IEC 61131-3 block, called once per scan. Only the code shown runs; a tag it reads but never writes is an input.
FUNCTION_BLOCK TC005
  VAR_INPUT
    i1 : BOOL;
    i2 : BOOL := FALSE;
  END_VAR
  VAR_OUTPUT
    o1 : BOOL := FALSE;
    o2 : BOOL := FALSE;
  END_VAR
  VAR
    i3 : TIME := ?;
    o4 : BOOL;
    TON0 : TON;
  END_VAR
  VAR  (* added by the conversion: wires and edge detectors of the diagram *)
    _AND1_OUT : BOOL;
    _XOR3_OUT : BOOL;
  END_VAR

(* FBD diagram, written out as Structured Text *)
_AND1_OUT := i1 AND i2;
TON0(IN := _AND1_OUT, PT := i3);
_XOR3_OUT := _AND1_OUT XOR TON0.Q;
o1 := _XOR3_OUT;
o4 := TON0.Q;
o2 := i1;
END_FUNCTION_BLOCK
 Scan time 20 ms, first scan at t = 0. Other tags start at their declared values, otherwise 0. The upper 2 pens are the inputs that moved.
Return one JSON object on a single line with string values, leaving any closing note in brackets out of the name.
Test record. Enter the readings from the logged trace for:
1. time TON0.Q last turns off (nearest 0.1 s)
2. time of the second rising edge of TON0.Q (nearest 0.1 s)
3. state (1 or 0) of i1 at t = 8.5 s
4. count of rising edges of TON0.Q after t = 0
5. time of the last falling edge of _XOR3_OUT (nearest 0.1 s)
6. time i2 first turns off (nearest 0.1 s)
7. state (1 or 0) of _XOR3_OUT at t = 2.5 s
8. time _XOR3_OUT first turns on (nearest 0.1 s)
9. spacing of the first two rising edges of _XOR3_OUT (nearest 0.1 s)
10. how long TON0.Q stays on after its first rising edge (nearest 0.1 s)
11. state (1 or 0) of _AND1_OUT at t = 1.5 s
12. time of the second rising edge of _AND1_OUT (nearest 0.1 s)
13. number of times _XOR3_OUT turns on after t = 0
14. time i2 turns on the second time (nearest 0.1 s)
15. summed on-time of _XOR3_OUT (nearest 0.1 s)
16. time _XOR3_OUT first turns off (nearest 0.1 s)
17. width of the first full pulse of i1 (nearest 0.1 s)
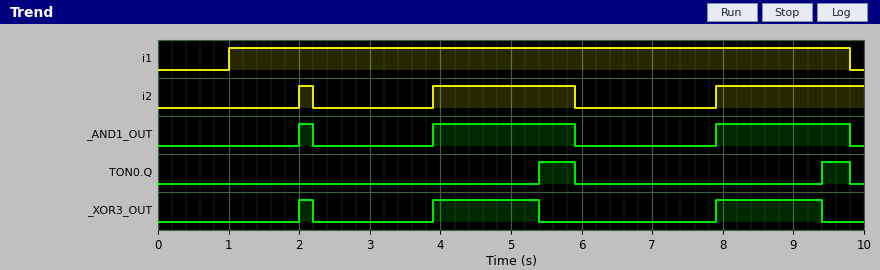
{"time TON0.Q last turns off": "9.8 s", "time of the second rising edge of TON0.Q": "9.4 s", "state (1 or 0) of i1 at t = 8.5 s": "1", "count of rising edges of TON0.Q after t = 0": "2", "time of the last falling edge of _XOR3_OUT": "9.4 s", "time i2 first turns off": "2.2 s", "state (1 or 0) of _XOR3_OUT at t = 2.5 s": "0", "time _XOR3_OUT first turns on": "2.0 s", "spacing of the first two rising edges of _XOR3_OUT": "1.9 s", "how long TON0.Q stays on after its first rising edge": "0.5 s", "state (1 or 0) of _AND1_OUT at t = 1.5 s": "0", "time of the second rising edge of _AND1_OUT": "3.9 s", "number of times _XOR3_OUT turns on after t = 0": "3", "time i2 turns on the second time": "3.9 s", "summed on-time of _XOR3_OUT": "3.2 s", "time _XOR3_OUT first turns off": "2.2 s", "width of the first full pulse of i1": "8.8 s"}
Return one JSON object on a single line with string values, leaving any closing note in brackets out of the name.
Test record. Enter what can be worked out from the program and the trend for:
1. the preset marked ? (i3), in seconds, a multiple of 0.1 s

{"the preset marked ? (i3), in seconds, a multiple of 0.1 s": "1.5 s"}
